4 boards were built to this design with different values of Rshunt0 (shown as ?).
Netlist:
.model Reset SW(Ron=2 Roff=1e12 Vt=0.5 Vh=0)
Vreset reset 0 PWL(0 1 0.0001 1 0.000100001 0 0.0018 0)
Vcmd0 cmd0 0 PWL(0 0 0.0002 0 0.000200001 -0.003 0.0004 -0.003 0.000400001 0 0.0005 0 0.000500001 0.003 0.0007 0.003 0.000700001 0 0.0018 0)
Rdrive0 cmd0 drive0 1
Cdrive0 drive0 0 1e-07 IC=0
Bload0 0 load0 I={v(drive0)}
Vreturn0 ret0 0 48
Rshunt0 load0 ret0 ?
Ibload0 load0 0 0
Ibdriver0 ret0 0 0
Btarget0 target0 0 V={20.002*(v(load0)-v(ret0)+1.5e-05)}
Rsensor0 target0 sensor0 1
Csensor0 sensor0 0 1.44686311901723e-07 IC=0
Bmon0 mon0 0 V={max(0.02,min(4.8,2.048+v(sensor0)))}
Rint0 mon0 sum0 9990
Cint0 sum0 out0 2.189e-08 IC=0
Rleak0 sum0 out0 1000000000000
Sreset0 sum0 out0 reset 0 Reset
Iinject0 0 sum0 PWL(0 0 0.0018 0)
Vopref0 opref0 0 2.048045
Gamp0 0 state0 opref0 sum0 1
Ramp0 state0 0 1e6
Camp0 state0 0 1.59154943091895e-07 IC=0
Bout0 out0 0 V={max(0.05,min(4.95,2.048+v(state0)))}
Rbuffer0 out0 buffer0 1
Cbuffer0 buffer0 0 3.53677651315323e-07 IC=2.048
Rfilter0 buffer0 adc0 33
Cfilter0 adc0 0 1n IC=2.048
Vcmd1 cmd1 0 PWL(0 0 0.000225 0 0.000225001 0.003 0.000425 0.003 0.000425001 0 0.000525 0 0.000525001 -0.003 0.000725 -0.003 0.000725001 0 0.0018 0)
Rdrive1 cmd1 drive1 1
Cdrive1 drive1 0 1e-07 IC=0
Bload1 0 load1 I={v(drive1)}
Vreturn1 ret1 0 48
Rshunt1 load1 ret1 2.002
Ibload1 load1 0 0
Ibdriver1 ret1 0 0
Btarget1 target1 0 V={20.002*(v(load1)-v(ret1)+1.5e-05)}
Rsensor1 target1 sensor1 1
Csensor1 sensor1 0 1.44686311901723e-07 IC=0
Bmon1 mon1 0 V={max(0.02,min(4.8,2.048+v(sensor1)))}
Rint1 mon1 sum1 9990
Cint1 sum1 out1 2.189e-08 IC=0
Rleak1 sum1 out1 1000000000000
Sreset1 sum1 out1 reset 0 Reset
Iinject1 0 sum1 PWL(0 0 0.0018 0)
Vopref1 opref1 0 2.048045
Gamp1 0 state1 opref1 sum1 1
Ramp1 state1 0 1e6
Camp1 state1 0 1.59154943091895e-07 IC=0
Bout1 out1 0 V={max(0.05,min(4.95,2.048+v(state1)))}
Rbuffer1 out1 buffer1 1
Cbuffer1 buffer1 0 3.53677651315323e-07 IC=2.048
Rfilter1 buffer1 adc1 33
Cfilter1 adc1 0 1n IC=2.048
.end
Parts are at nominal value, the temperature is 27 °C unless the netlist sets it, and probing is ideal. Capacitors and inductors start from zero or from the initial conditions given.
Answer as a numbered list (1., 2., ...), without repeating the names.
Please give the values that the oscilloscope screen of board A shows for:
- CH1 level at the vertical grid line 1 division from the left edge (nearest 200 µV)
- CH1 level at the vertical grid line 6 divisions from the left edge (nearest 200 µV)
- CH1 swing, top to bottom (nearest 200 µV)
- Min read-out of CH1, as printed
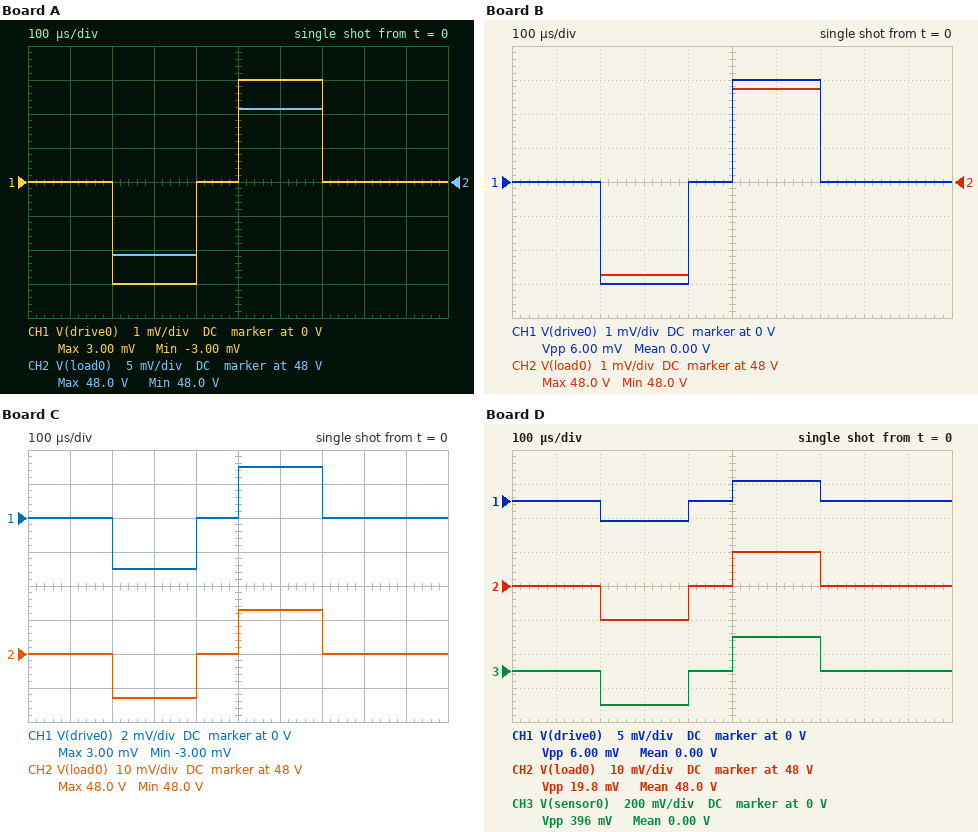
1. 0 V
2. 3.0 mV
3. 6.0 mV
4. -3.00 mV
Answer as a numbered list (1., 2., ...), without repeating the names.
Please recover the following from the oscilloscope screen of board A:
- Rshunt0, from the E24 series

1. 3.6 Ω
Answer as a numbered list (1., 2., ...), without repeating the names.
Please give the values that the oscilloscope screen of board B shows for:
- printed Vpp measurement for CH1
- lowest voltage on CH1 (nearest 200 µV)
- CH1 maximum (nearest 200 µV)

1. 6.00 mV
2. -3.0 mV
3. 3.0 mV
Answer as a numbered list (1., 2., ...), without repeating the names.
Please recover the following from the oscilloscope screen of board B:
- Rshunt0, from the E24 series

1. 0.91 Ω
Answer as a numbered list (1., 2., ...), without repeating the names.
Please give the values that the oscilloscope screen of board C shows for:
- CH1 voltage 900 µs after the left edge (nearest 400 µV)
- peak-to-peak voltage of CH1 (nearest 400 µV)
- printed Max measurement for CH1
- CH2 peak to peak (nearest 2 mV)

1. 0 V
2. 6.0 mV
3. 3.00 mV
4. 26 mV
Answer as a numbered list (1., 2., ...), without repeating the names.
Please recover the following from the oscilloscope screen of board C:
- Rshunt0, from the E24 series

1. 4.3 Ω
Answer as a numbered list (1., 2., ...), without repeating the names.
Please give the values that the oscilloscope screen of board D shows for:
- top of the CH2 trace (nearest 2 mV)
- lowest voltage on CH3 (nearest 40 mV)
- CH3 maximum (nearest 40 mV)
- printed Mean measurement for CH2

1. 48.010 V
2. -200 mV
3. 200 mV
4. 48.0 V
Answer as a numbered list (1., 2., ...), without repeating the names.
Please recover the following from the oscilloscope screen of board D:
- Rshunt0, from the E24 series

1. 3.3 Ω
